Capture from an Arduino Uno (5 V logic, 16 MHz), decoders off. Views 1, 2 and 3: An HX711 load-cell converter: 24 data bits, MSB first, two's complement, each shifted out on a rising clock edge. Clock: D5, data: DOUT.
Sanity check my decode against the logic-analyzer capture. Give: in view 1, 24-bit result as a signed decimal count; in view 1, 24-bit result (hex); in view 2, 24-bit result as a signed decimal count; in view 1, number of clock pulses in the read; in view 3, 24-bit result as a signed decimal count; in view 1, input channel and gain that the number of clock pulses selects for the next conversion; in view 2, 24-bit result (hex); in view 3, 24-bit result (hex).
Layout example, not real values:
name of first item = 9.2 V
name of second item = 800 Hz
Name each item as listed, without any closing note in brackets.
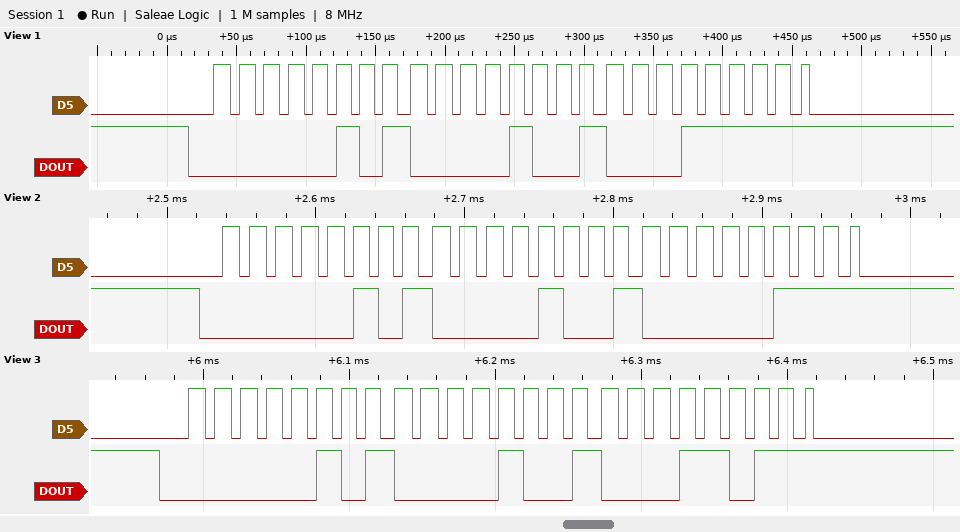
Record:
in view 1, 24-bit result as a signed decimal count = 330015
in view 1, 24-bit result = 0x05091F
in view 2, 24-bit result as a signed decimal count = 329991
in view 1, number of clock pulses in the read = 25
in view 3, 24-bit result as a signed decimal count = 330011
in view 1, input channel and gain that the number of clock pulses selects for the next conversion = channel A, gain 128
in view 2, 24-bit result = 0x050907
in view 3, 24-bit result = 0x05091B
